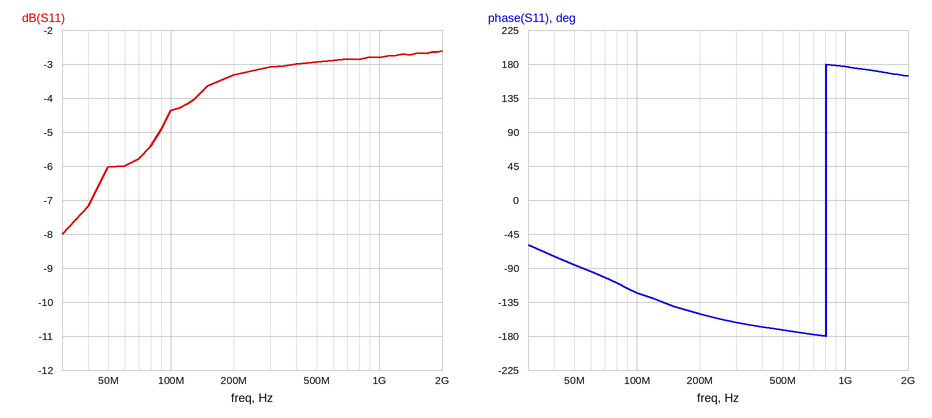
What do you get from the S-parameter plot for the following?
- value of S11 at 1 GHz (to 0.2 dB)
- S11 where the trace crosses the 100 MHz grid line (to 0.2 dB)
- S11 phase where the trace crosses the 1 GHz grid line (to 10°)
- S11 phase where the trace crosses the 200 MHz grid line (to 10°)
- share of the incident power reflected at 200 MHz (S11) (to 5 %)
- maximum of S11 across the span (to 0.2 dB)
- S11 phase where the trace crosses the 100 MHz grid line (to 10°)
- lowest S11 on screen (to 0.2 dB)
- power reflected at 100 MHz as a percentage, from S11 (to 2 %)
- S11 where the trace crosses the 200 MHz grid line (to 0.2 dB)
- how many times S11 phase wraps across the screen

-2.8 dB
-4.4 dB
180°
-150°
45 %
-2.6 dB
-120°
-8.0 dB
36 %
-3.4 dB
1
